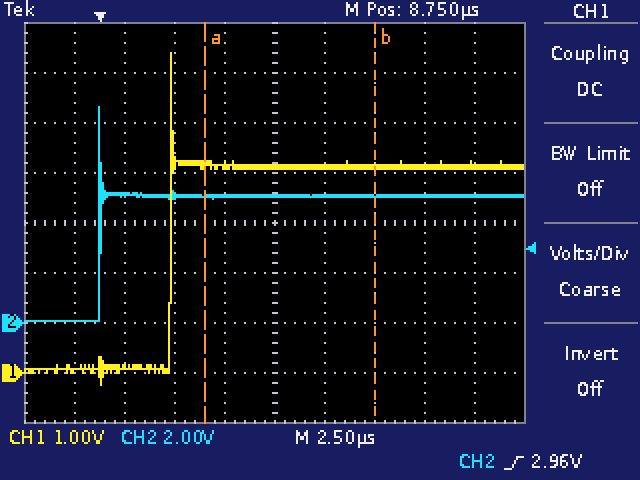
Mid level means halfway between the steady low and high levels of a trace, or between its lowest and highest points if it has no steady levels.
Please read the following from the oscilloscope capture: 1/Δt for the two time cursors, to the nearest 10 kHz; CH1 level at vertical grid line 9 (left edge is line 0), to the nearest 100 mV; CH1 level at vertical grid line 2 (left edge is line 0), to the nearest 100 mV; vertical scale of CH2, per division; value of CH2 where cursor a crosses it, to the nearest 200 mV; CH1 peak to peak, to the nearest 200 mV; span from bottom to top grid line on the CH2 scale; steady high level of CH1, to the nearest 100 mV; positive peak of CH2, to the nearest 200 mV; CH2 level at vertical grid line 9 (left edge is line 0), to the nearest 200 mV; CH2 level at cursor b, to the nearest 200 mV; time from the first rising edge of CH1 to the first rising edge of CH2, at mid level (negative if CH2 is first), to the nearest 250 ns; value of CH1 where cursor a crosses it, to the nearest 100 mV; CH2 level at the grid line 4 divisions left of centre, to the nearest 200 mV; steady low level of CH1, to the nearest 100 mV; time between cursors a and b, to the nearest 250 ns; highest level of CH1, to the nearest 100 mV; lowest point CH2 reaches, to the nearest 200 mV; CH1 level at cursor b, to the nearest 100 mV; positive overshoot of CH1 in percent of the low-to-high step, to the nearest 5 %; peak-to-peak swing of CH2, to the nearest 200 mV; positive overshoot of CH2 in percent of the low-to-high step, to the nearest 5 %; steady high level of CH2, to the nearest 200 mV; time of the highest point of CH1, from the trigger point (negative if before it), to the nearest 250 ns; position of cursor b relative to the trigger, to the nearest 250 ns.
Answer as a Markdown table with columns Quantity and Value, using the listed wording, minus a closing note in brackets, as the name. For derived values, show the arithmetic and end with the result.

| Quantity | Value |
|---|---|
| 1/Δt for the two time cursors, to the nearest 10 kHz | 1 / 8.50 µs ≈ 120 kHz |
| CH1 level at vertical grid line 9 (left edge is line 0), to the nearest 100 mV | 4.2 V |
| CH1 level at vertical grid line 2 (left edge is line 0), to the nearest 100 mV | 100 mV |
| vertical scale of CH2, per division | 2 V |
| value of CH2 where cursor a crosses it, to the nearest 200 mV | 5.0 V |
| CH1 peak to peak, to the nearest 200 mV | 6.6 V |
| span from bottom to top grid line on the CH2 scale | 16 V |
| steady high level of CH1, to the nearest 100 mV | 4.1 V |
| positive peak of CH2, to the nearest 200 mV | 8.6 V |
| CH2 level at vertical grid line 9 (left edge is line 0), to the nearest 200 mV | 5.0 V |
| CH2 level at cursor b, to the nearest 200 mV | 5.0 V |
| time from the first rising edge of CH1 to the first rising edge of CH2, at mid level (negative if CH2 is first), to the nearest 250 ns | -3.50 µs |
| value of CH1 where cursor a crosses it, to the nearest 100 mV | 4.2 V |
| CH2 level at the grid line 4 divisions left of centre, to the nearest 200 mV | 0.0 V |
| steady low level of CH1, to the nearest 100 mV | 100 mV |
| time between cursors a and b, to the nearest 250 ns | 8.50 µs |
| highest level of CH1, to the nearest 100 mV | 6.4 V |
| lowest point CH2 reaches, to the nearest 200 mV | 0.0 V |
| CH1 level at cursor b, to the nearest 100 mV | 4.1 V |
| positive overshoot of CH1 in percent of the low-to-high step, to the nearest 5 % | 55 % |
| peak-to-peak swing of CH2, to the nearest 200 mV | 8.6 V − (0.0 V) = 8.6 V |
| positive overshoot of CH2 in percent of the low-to-high step, to the nearest 5 % | 70 % |
| steady high level of CH2, to the nearest 200 mV | 5.0 V |
| time of the highest point of CH1, from the trigger point (negative if before it), to the nearest 250 ns | +3.50 µs |
| position of cursor b relative to the trigger, to the nearest 250 ns | +13.75 µs |
